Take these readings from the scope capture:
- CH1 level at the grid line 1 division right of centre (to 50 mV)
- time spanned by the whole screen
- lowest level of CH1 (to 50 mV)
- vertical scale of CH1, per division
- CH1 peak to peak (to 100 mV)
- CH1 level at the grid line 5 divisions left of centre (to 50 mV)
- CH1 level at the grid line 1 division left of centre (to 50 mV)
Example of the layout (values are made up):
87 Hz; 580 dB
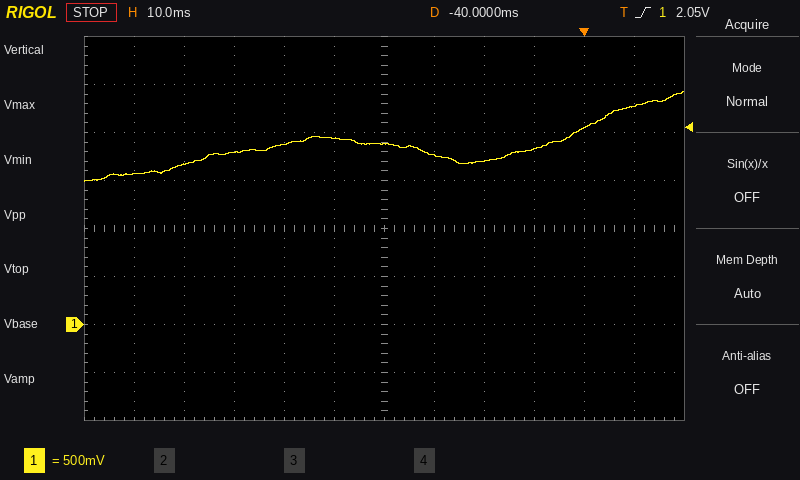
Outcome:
1.75 V; 120 ms; 1.50 V; 500 mV; 900 mV; 1.55 V; 1.95 V
